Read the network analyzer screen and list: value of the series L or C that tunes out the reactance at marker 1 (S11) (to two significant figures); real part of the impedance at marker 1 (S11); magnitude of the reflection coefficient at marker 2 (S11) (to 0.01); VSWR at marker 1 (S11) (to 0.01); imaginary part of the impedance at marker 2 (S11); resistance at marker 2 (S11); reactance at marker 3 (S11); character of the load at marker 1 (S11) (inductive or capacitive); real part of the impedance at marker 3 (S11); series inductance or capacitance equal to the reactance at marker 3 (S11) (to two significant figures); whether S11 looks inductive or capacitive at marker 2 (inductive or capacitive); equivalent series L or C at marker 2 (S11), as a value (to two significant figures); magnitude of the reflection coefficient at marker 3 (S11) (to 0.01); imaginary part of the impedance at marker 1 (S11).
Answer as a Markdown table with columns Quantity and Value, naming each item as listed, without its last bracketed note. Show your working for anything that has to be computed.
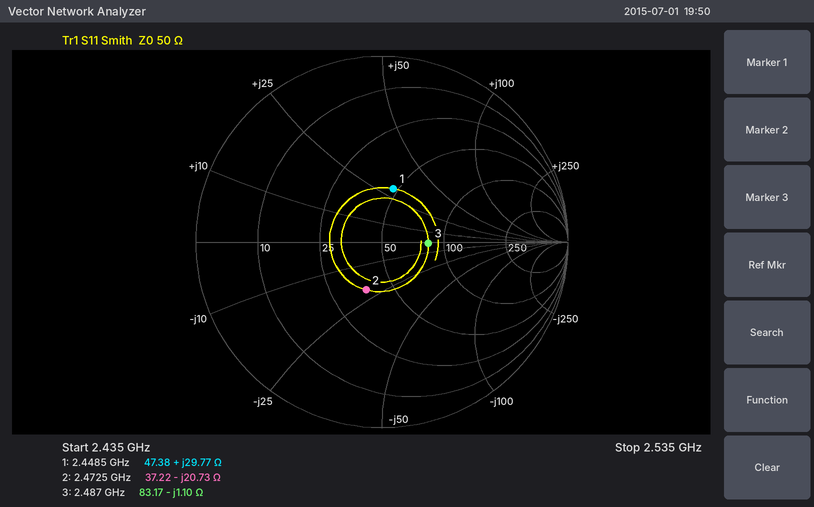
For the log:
| Quantity | Value |
|---|---|
| value of the series L or C that tunes out the reactance at marker 1 (S11) | C = 1/(2π × 2.4485 GHz × 29.77 Ω) ≈ 2.2 pF |
| real part of the impedance at marker 1 | 47.38 Ω |
| magnitude of the reflection coefficient at marker 2 (S11) | 0.27 |
| VSWR at marker 1 (S11) | 1.83 |
| imaginary part of the impedance at marker 2 | -20.73 Ω |
| resistance at marker 2 | 37.22 Ω |
| reactance at marker 3 | -1.10 Ω |
| character of the load at marker 1 (S11) | inductive |
| real part of the impedance at marker 3 | 83.17 Ω |
| series inductance or capacitance equal to the reactance at marker 3 (S11) | C = 1/(2π × 2.487 GHz × 1.1 Ω) ≈ 58 pF |
| whether S11 looks inductive or capacitive at marker 2 | capacitive |
| equivalent series L or C at marker 2 (S11), as a value | C = 1/(2π × 2.4725 GHz × 20.73 Ω) ≈ 3.1 pF |
| magnitude of the reflection coefficient at marker 3 (S11) | 0.25 |
| imaginary part of the impedance at marker 1 | +29.77 Ω |
